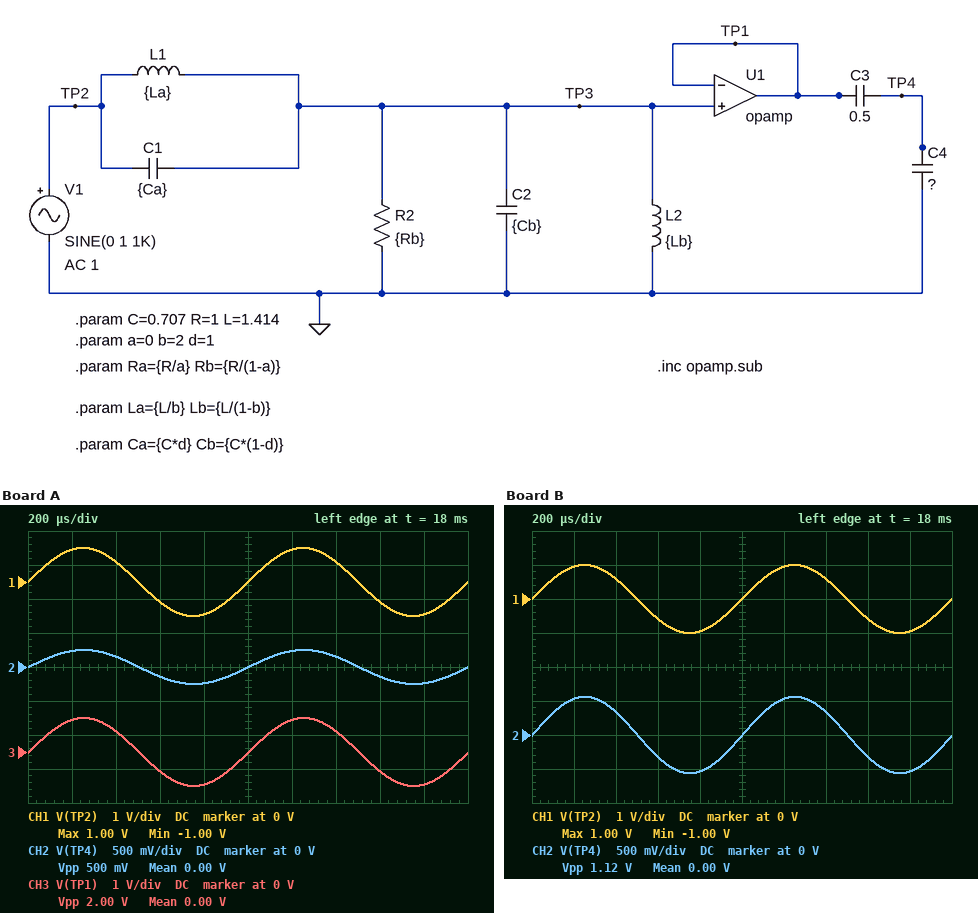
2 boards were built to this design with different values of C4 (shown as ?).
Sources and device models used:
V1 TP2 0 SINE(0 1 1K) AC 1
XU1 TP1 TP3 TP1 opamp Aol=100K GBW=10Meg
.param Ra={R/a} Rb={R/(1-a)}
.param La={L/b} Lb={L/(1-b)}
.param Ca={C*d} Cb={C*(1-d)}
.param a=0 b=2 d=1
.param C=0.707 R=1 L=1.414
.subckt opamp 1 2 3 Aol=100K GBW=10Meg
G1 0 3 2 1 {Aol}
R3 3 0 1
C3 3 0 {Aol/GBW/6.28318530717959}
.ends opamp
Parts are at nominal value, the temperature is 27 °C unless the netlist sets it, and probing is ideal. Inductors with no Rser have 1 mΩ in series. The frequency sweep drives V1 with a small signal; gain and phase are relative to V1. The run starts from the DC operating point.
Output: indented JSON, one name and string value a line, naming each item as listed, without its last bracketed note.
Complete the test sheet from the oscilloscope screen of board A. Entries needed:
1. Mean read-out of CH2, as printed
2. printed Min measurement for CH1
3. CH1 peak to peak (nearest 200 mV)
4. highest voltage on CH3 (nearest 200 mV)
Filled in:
{
  "Mean read-out of CH2, as printed": "0.00 V",
  "printed Min measurement for CH1": "-1.00 V",
  "CH1 peak to peak": "2.0 V",
  "highest voltage on CH3": "1.0 V"
}
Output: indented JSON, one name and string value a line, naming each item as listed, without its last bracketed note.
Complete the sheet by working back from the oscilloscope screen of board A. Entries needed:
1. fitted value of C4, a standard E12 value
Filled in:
{
  "fitted value of C4, a standard E12 value": "1.5 F"
}
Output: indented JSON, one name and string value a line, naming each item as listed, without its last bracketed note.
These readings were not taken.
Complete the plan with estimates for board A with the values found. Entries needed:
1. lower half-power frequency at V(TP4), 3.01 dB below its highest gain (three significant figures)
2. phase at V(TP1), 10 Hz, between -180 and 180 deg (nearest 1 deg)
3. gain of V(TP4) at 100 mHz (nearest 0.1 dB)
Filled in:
{
  "lower half-power frequency at V(TP4), 3.01 dB below its highest gain": "417 µHz",
  "phase at V(TP1), 10 Hz, between -180 and 180 deg": "1 deg",
  "gain of V(TP4) at 100 mHz": "-8.6 dB"
}
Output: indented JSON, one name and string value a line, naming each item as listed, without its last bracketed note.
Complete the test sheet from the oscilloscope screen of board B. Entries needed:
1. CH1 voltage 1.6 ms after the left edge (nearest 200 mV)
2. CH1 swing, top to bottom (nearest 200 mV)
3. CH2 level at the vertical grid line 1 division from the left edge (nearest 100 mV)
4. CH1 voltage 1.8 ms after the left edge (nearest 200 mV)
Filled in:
{
  "CH1 voltage 1.6 ms after the left edge": "-600 mV",
  "CH1 swing, top to bottom": "2.0 V",
  "CH2 level at the vertical grid line 1 division from the left edge": "500 mV",
  "CH1 voltage 1.8 ms after the left edge": "-1.0 V"
}
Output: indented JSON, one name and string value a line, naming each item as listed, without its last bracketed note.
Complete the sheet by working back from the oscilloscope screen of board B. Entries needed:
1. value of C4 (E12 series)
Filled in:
{
  "value of C4": "390 mF"
}
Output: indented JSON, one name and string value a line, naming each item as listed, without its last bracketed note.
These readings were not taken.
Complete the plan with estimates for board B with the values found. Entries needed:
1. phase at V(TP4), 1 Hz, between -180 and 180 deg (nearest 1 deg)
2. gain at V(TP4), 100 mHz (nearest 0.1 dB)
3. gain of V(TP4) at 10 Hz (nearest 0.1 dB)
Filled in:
{
  "phase at V(TP4), 1 Hz, between -180 and 180 deg": "13 deg",
  "gain at V(TP4), 100 mHz": "-1.6 dB",
  "gain of V(TP4) at 10 Hz": "-5.0 dB"
}
